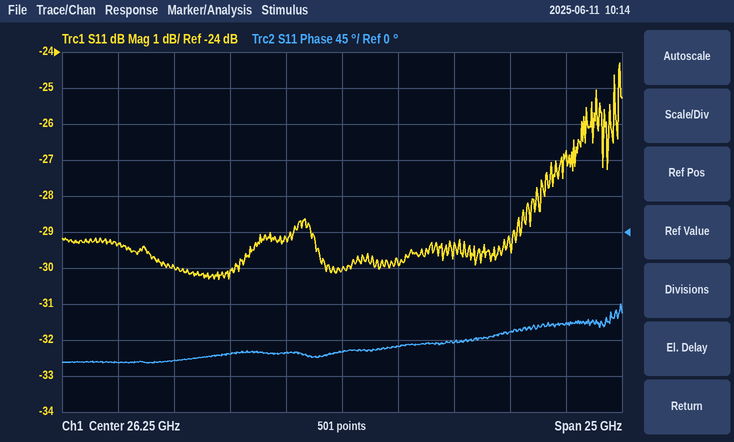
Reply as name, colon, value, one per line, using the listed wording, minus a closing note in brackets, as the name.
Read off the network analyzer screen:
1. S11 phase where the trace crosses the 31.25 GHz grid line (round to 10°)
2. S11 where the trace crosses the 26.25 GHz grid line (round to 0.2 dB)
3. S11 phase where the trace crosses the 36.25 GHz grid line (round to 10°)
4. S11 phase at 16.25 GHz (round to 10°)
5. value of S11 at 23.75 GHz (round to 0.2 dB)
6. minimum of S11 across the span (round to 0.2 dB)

S11 phase where the trace crosses the 31.25 GHz grid line: -140°
S11 where the trace crosses the 26.25 GHz grid line: -30.0 dB
S11 phase where the trace crosses the 36.25 GHz grid line: -110°
S11 phase at 16.25 GHz: -160°
value of S11 at 23.75 GHz: -29.2 dB
minimum of S11 across the span: -30.4 dB
